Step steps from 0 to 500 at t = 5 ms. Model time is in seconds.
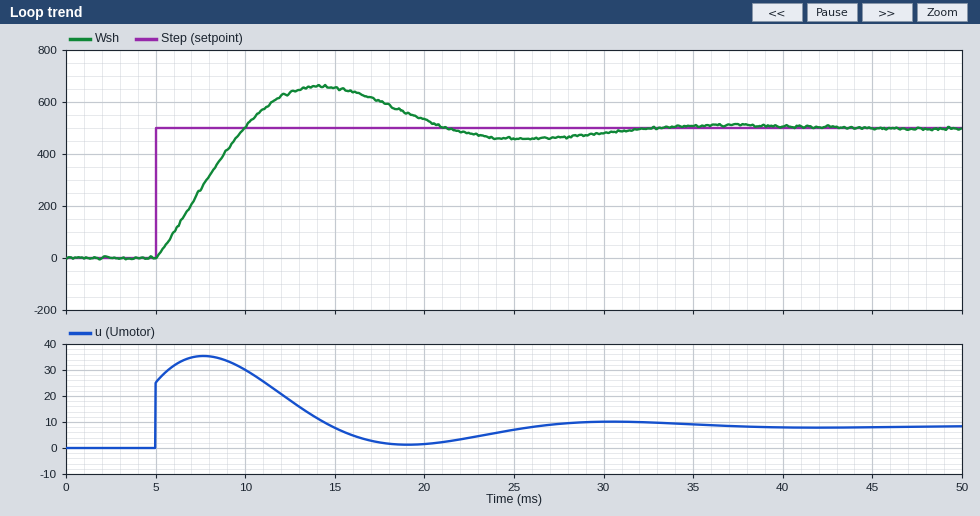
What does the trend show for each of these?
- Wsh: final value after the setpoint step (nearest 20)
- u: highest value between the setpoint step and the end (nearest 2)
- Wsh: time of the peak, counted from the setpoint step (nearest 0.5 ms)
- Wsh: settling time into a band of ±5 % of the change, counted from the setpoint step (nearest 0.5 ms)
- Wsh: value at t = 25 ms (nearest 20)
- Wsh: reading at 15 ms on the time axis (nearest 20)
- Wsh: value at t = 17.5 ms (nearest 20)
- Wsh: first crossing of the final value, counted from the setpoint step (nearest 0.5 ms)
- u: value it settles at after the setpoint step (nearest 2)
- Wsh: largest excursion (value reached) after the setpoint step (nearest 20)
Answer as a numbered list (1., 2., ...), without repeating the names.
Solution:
1. 500
2. 36
3. 9.0 ms
4. 24.0 ms
5. 460
6. 660
7. 600
8. 5.0 ms
9. 8
10. 660
